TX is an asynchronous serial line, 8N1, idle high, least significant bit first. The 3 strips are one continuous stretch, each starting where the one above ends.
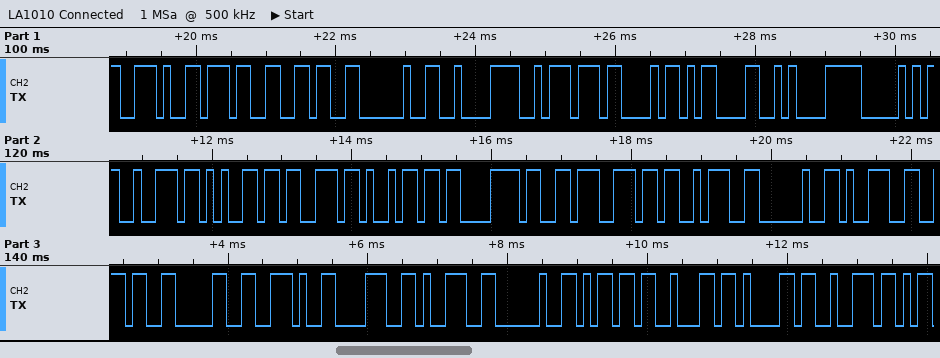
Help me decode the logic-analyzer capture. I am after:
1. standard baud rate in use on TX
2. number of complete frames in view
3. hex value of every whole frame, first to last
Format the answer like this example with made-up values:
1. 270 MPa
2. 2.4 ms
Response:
1. 9600 baud
2. 30
3. 2E 37 36 20 C2 BA 43 0D 0A 50 72 65 73 69 C3 B3 6E 3A 20 39 36 30 2E 38 39 20 6D 62 61 72
